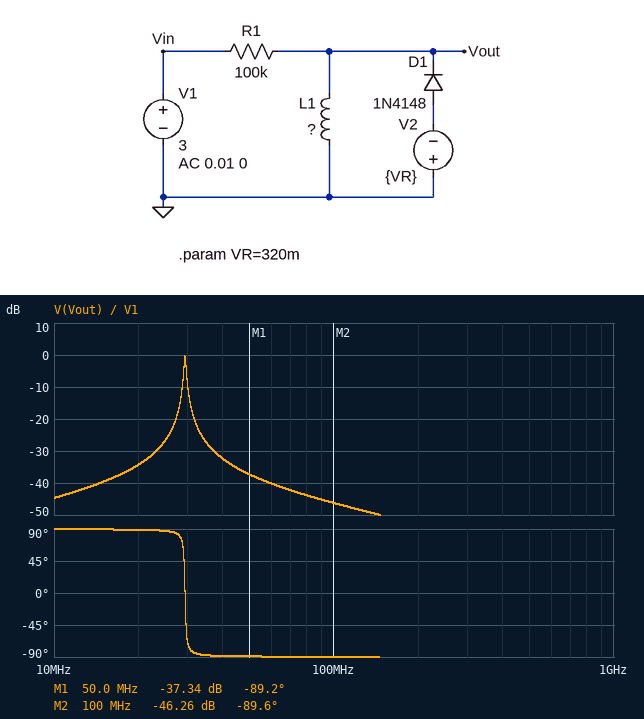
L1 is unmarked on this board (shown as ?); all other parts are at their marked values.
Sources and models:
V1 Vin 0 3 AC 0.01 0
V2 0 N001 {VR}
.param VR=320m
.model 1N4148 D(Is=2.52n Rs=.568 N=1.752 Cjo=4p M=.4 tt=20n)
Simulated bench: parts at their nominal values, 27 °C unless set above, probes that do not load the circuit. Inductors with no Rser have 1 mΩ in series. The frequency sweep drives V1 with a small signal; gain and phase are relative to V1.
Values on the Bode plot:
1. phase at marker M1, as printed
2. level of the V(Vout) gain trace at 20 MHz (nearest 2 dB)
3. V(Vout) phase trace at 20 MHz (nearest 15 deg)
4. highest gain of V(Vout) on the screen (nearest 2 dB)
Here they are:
-89.2 deg
-34 dB
90 deg
0 dB
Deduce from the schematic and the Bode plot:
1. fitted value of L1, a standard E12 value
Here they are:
8.2 µH
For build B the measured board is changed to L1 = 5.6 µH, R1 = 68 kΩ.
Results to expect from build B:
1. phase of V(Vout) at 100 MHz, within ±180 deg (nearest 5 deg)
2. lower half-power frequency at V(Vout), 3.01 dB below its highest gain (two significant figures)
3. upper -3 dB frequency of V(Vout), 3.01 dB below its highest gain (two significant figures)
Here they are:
-90 deg
35 MHz
36 MHz
